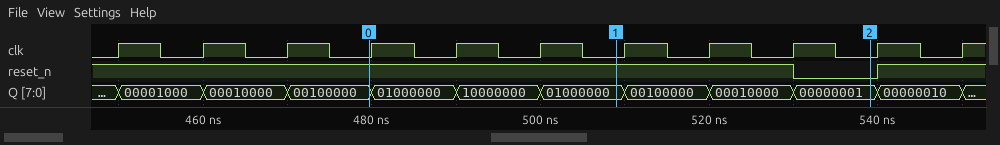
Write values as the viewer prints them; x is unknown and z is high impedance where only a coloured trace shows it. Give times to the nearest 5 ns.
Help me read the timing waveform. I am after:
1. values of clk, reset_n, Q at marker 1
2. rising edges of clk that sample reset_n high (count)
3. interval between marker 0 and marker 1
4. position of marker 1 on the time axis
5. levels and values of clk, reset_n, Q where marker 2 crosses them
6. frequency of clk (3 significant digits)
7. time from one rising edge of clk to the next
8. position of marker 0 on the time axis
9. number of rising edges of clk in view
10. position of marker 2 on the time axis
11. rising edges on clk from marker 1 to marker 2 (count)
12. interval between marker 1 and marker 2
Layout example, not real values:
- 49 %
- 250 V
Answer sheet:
- clk=0, reset_n=1, Q=01000000
- 10
- 30 ns
- 510 ns
- clk=0, reset_n=0, Q=00000001
- 100 MHz
- 10 ns
- 480 ns
- 11
- 540 ns
- 3
- 30 ns
